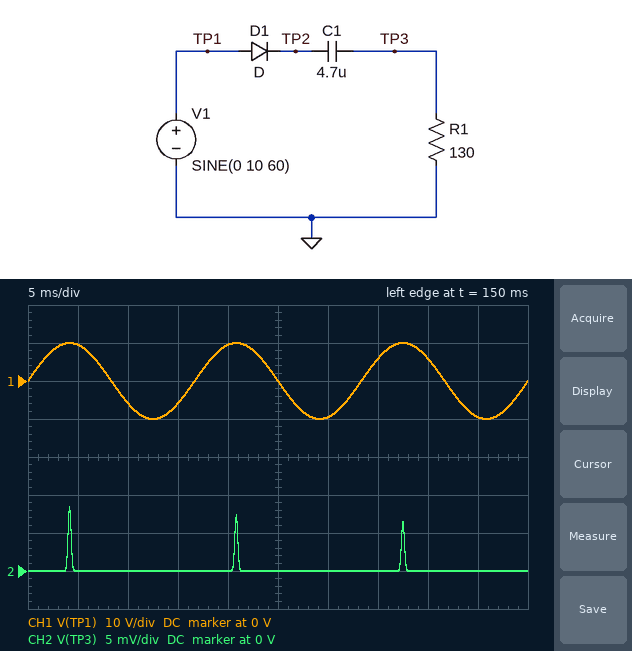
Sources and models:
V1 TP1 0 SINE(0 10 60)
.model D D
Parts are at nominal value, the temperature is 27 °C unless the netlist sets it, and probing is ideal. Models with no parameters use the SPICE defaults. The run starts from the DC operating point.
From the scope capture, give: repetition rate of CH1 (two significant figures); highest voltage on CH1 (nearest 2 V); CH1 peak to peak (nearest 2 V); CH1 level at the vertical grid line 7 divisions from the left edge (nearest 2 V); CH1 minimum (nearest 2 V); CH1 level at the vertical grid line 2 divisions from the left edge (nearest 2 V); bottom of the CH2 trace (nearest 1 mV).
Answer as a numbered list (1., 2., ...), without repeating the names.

1. 60 Hz
2. 10 V
3. 20 V
4. 6 V
5. -10 V
6. -6 V
7. 0 V
